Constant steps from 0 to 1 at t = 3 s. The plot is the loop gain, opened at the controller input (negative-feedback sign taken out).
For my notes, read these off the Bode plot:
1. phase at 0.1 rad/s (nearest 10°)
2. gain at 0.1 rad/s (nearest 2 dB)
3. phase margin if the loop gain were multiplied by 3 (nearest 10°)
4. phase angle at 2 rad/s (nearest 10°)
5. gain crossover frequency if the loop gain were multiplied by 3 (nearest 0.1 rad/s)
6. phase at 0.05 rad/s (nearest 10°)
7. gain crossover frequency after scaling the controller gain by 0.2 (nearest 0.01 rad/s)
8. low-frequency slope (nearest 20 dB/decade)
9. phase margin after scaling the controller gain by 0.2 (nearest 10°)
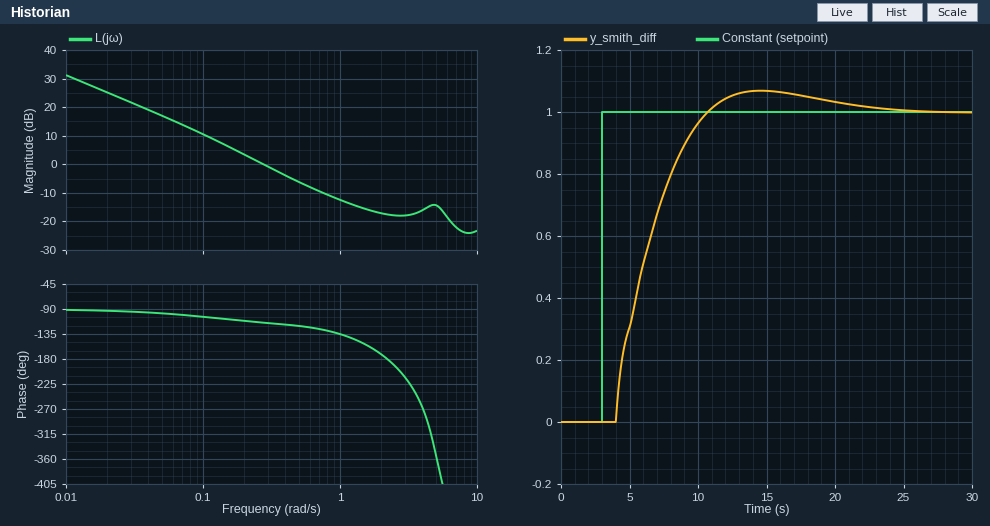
-100°
10 dB
50°
-170°
0.7 rad/s
-100°
0.07 rad/s
-20 dB/decade
80°
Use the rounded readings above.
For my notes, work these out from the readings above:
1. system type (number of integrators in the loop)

1
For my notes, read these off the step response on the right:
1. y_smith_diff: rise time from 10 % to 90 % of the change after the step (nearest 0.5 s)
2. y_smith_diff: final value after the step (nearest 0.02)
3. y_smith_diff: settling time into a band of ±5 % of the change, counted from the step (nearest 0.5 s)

5.0 s
1.00
15.0 s
